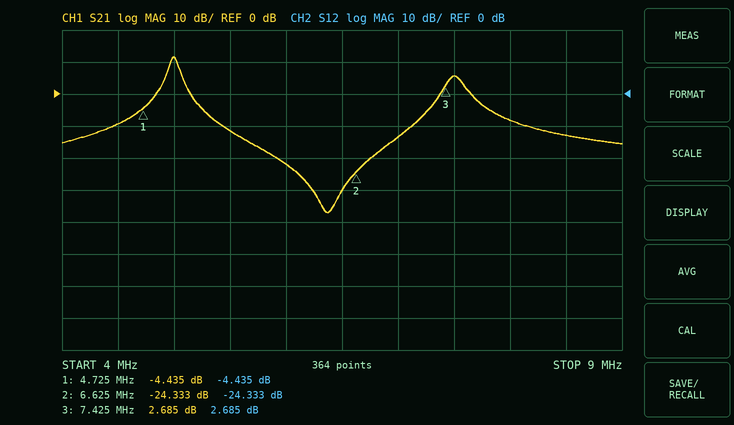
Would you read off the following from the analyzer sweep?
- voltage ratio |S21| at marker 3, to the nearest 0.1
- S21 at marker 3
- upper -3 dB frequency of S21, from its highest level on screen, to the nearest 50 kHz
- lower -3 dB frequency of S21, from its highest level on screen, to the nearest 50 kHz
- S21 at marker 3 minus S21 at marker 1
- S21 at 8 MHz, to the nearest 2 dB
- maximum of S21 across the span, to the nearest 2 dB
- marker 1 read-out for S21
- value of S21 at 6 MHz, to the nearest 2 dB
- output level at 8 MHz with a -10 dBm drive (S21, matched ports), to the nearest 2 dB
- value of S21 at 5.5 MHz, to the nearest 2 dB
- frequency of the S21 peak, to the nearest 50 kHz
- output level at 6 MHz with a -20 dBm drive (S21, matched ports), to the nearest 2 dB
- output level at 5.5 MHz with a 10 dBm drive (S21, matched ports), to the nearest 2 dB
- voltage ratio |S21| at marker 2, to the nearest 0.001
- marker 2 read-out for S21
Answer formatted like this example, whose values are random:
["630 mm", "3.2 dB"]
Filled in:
["1.4", "2.685 dB", "5.05 MHz", "4.95 MHz", "7.120 dB", "-8 dB", "12 dB", "-4.435 dB", "-22 dB", "-18 dBm", "-12 dB", "5.00 MHz", "-42 dBm", "-2 dBm", "0.061", "-24.333 dB"]
